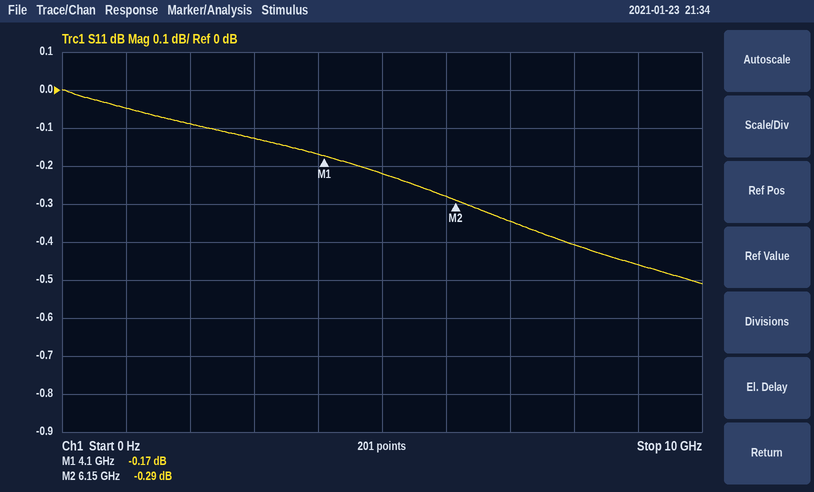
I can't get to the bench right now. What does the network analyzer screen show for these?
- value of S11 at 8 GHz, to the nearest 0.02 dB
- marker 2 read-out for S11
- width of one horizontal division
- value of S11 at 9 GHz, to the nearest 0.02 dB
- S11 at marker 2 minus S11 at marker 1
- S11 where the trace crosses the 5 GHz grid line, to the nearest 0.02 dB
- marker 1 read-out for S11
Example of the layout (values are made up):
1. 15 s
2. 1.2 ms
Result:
1. -0.40 dB
2. -0.29 dB
3. 1 GHz
4. -0.46 dB
5. -0.12 dB
6. -0.22 dB
7. -0.17 dB
